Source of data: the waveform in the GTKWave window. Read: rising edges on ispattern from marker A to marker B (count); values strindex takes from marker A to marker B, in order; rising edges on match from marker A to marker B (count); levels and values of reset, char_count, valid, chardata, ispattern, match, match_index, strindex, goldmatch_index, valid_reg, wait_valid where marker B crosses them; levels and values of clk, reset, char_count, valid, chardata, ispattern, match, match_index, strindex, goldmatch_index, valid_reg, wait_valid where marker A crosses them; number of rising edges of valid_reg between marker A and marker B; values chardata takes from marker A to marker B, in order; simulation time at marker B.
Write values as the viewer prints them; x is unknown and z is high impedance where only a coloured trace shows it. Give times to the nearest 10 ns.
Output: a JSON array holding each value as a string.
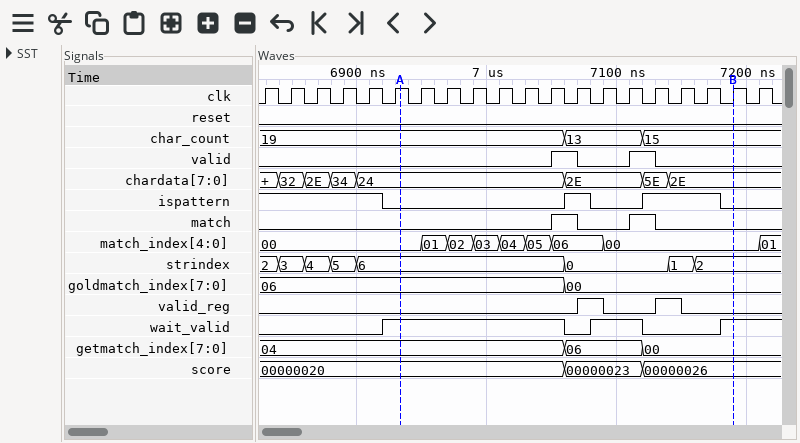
["2", "6, 0, 1, 2", "2", "reset=0, char_count=15, valid=0, chardata=2E, ispattern=0, match=0, match_index=00, strindex=2, goldmatch_index=00, valid_reg=0, wait_valid=1", "clk=1, reset=0, char_count=19, valid=0, chardata=24, ispattern=0, match=0, match_index=00, strindex=6, goldmatch_index=06, valid_reg=0, wait_valid=1", "2", "24, 2E, 5E, 2E", "7190 ns"]
